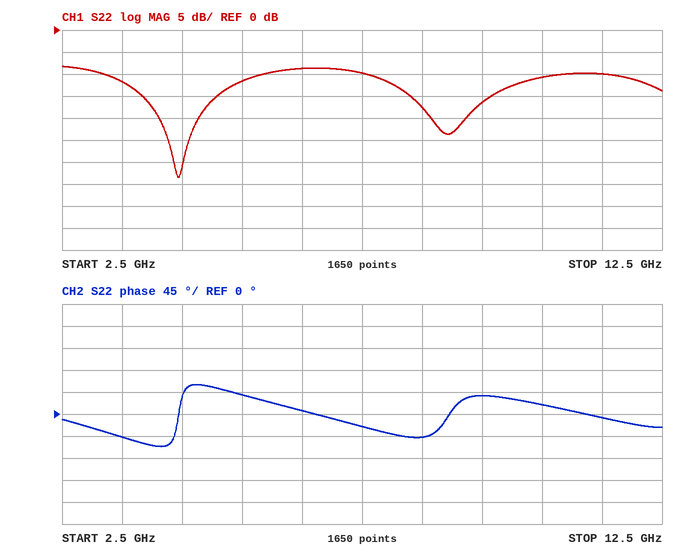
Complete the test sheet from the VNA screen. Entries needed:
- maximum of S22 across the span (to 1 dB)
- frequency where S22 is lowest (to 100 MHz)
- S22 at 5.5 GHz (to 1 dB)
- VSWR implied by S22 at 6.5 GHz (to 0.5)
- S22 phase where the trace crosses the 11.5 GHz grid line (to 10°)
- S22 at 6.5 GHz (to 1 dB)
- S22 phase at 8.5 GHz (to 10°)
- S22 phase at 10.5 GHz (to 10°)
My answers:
-8 dB
4.4 GHz
-12 dB
2.0
-10°
-9 dB
-50°
20°
